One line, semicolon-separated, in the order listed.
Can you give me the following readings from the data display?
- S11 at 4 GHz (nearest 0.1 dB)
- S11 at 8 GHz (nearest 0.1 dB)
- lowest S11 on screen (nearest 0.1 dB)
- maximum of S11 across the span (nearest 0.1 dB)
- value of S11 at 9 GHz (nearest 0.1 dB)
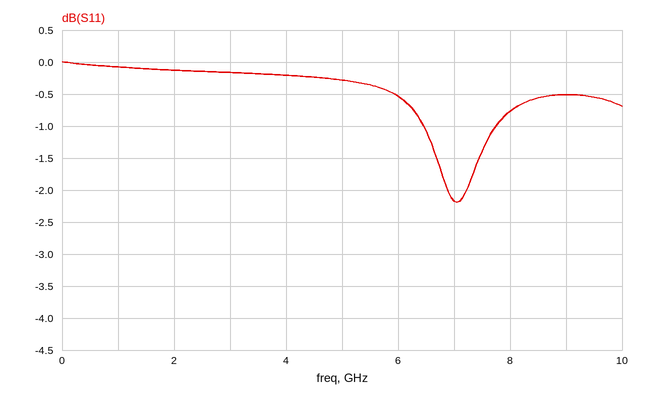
-0.2 dB; -0.8 dB; -2.2 dB; 0.0 dB; -0.5 dB
